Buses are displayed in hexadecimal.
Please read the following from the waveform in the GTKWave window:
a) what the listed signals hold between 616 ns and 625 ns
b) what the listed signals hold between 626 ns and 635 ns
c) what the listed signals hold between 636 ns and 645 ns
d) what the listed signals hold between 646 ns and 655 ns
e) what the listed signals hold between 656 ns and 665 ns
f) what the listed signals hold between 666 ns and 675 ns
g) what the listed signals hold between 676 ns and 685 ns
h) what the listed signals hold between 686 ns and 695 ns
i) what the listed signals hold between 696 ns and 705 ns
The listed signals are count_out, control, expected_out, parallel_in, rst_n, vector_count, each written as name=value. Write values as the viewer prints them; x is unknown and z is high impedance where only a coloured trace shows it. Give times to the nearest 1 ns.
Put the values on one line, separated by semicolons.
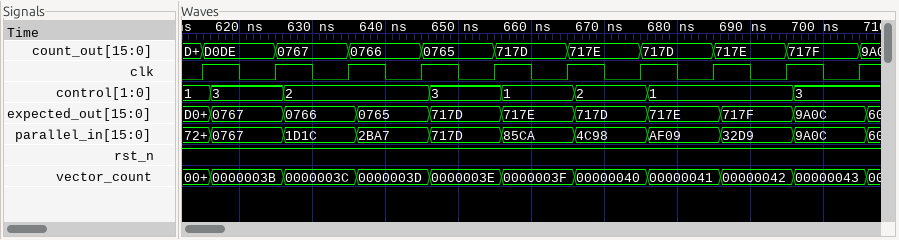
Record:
count_out=D0DE, control=3, expected_out=0767, parallel_in=0767, rst_n=1, vector_count=0000003B; count_out=0767, control=2, expected_out=0766, parallel_in=1D1C, rst_n=1, vector_count=0000003C; count_out=0766, control=2, expected_out=0765, parallel_in=2BA7, rst_n=1, vector_count=0000003D; count_out=0765, control=3, expected_out=717D, parallel_in=717D, rst_n=1, vector_count=0000003E; count_out=717D, control=1, expected_out=717E, parallel_in=85CA, rst_n=1, vector_count=0000003F; count_out=717E, control=2, expected_out=717D, parallel_in=4C98, rst_n=1, vector_count=00000040; count_out=717D, control=1, expected_out=717E, parallel_in=AF09, rst_n=1, vector_count=00000041; count_out=717E, control=1, expected_out=717F, parallel_in=32D9, rst_n=1, vector_count=00000042; count_out=717F, control=3, expected_out=9A0C, parallel_in=9A0C, rst_n=1, vector_count=00000043
